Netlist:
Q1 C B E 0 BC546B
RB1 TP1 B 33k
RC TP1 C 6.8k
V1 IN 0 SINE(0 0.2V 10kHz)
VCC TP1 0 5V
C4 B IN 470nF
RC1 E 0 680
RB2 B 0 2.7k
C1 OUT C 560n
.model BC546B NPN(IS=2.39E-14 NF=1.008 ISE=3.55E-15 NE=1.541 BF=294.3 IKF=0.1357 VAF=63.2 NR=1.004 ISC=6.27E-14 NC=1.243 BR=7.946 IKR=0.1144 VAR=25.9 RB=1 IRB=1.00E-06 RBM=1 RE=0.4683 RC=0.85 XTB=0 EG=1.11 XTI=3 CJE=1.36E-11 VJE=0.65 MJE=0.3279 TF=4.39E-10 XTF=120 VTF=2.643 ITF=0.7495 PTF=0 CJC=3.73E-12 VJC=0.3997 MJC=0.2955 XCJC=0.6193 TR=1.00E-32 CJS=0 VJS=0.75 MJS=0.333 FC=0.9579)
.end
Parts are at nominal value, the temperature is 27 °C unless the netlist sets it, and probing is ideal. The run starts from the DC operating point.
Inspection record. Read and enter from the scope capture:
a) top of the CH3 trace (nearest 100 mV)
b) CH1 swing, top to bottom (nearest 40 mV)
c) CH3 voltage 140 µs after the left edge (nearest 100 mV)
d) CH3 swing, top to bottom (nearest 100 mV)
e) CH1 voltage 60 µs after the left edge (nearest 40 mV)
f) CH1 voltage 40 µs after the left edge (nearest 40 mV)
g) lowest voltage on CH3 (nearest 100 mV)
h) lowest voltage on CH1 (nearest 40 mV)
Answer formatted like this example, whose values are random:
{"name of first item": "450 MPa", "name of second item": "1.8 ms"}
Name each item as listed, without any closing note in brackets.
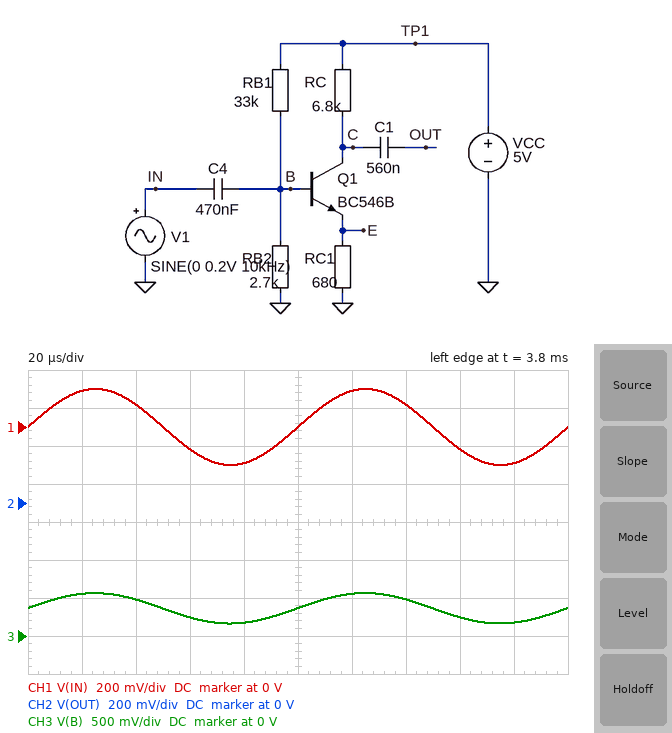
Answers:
{"top of the CH3 trace": "600 mV", "CH1 swing, top to bottom": "400 mV", "CH3 voltage 140 µs after the left edge": "500 mV", "CH3 swing, top to bottom": "400 mV", "CH1 voltage 60 µs after the left edge": "-120 mV", "CH1 voltage 40 µs after the left edge": "120 mV", "lowest voltage on CH3": "200 mV", "lowest voltage on CH1": "-200 mV"}
